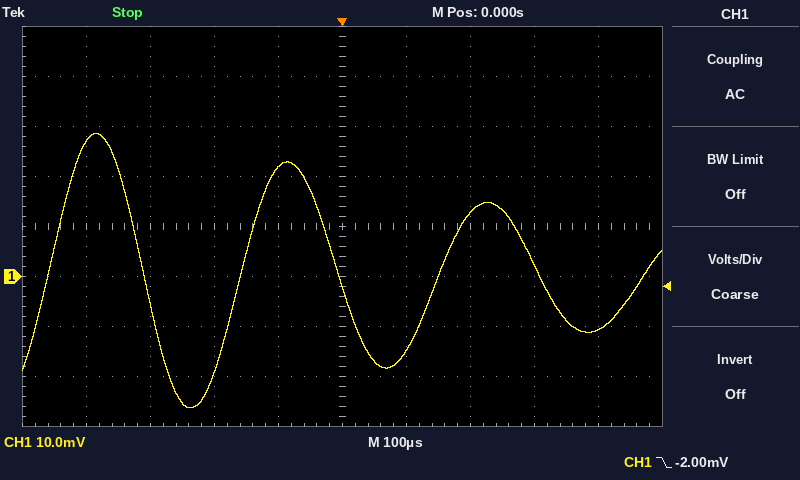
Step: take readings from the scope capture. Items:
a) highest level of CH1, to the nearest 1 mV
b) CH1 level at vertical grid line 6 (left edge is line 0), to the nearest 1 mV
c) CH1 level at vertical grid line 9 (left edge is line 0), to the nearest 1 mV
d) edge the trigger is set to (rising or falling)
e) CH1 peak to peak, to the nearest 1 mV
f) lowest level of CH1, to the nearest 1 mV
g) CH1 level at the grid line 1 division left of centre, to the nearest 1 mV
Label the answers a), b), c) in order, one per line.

a) 29 mV
b) -15 mV
c) -11 mV
d) falling
e) 55 mV
f) -26 mV
g) 22 mV
